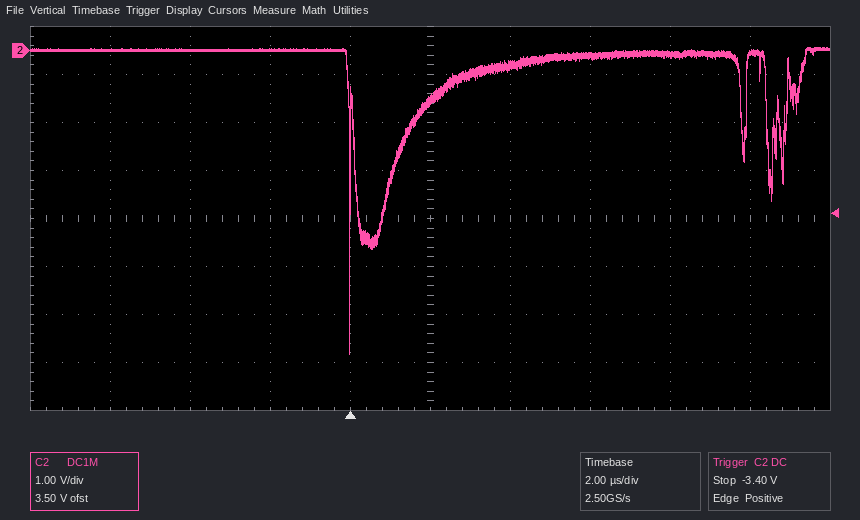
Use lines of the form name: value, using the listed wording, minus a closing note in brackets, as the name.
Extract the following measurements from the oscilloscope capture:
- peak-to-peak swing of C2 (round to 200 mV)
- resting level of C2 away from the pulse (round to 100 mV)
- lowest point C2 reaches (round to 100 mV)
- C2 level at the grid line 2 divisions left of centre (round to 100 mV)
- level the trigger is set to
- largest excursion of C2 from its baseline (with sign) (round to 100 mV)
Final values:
peak-to-peak swing of C2: 6.4 V
resting level of C2 away from the pulse: 0.0 V
lowest point C2 reaches: -6.3 V
C2 level at the grid line 2 divisions left of centre: 0.0 V
level the trigger is set to: -3.40 V
largest excursion of C2 from its baseline (with sign): -6.3 V
